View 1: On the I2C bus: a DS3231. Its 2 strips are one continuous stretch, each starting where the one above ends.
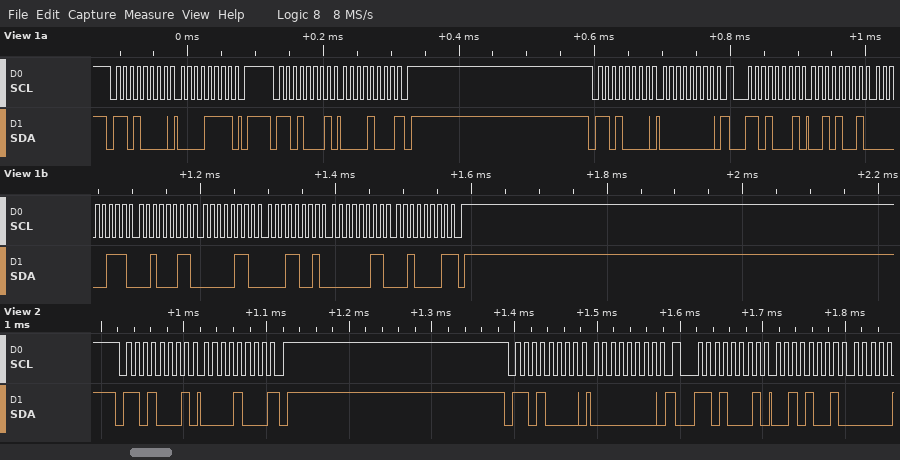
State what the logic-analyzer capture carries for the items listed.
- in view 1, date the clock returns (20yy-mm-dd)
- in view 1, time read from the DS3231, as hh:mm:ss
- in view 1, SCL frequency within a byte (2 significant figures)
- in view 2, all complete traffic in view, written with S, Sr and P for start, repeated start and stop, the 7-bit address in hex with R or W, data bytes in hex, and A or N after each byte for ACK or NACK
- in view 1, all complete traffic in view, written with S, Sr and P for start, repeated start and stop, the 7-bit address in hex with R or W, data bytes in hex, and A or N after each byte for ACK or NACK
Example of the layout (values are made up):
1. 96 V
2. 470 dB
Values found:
1. 2021-03-19
2. 23:07:29
3. 100 kHz
4. S 68R A 08 N P S 68W A 00 A Sr 68R A 29 A
5. S 68W A 0F A P S 68R A 08 N P S 68W A 00 A Sr 68R A 29 A 07 A 23 A 06 A 19 A 03 A 21 N P
